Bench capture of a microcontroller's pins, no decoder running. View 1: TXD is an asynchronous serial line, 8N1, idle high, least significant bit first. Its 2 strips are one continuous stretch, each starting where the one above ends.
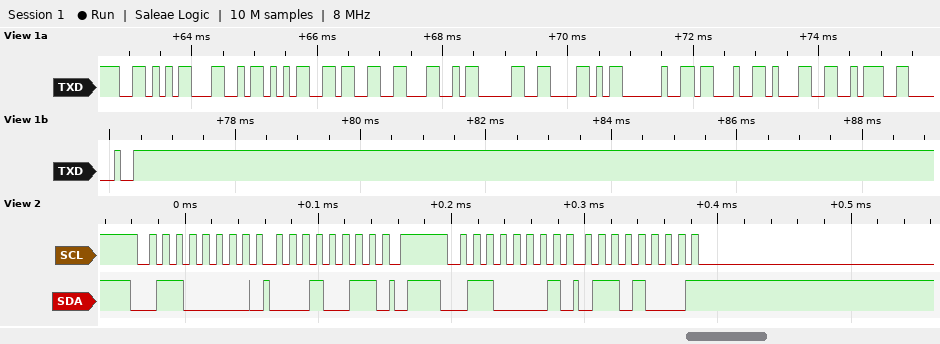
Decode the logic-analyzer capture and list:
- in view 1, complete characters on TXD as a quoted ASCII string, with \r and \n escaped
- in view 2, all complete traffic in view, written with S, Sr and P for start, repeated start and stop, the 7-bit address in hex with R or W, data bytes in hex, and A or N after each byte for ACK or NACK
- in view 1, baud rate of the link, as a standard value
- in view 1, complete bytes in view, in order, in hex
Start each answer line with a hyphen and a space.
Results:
- "VL53L0X #1: "
- S 30W A 13 A P S 30R A 68 N
- 9600 baud
- 56 4C 35 33 4C 30 58 20 23 31 3A 20
